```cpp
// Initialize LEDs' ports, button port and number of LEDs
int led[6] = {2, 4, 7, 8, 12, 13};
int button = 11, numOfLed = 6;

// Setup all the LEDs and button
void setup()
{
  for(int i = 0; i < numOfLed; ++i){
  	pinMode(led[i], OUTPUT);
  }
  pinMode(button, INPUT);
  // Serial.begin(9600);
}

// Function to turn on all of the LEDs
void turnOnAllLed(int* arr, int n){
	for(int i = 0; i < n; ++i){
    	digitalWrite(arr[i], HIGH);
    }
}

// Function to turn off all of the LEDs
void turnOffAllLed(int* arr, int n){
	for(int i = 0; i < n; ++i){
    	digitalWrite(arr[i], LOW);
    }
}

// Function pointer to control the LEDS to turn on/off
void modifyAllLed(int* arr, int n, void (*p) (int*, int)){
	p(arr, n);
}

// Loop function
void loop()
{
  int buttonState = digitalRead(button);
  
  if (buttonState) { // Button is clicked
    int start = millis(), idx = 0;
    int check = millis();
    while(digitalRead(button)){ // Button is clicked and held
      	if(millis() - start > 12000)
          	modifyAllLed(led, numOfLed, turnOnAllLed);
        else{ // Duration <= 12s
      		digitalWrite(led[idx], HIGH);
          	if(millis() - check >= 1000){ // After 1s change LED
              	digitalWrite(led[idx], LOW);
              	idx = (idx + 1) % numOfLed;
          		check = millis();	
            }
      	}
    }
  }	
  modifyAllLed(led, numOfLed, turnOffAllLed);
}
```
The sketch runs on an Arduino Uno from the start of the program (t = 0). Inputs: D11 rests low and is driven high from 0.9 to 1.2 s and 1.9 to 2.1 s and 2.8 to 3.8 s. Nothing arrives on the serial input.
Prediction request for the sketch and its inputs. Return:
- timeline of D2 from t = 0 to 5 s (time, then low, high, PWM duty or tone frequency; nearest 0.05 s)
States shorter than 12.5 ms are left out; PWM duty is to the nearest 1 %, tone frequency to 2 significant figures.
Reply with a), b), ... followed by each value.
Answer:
a) 0 s low; 0.9 s high; 1.2 s low; 1.9 s high; 2.1 s low; 2.8 s high; 3.8 s low
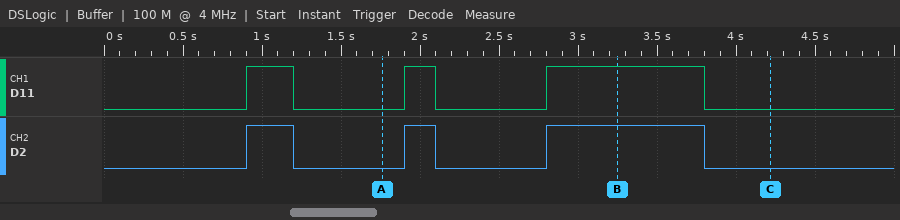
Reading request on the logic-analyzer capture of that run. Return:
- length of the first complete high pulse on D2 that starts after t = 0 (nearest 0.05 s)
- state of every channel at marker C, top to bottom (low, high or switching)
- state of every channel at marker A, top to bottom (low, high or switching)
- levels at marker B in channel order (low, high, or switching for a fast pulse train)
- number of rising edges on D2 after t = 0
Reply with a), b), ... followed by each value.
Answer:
a) 0.30 s
b) D11 low, D2 low
c) D11 low, D2 low
d) D11 high, D2 high
e) 3
